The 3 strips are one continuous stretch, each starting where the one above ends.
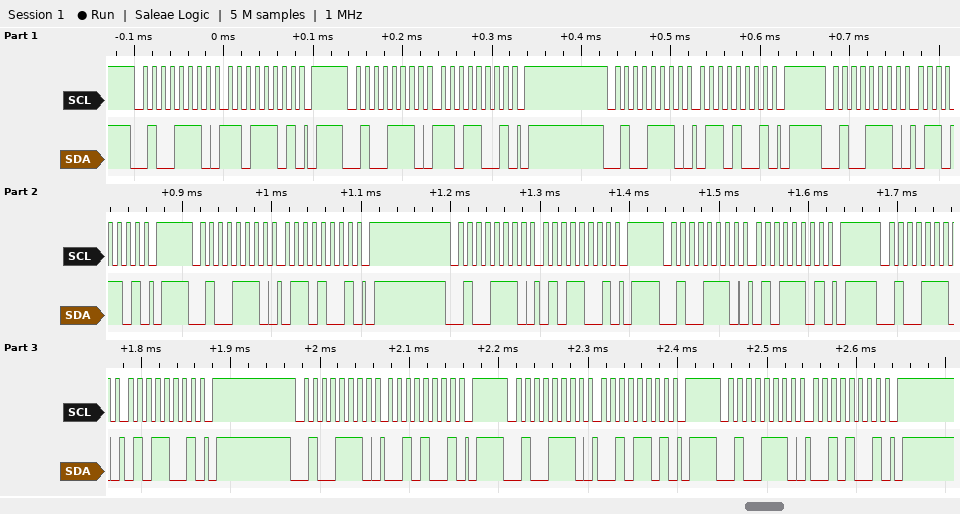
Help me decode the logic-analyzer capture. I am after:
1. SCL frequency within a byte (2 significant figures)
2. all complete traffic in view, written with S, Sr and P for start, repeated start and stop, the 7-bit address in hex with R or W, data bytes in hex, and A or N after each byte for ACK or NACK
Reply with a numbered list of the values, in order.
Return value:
1. 100 kHz
2. S 27W A DD A P S 27W A D9 A P S 27W A 69 A P S 27W A 6D A P S 27W A 69 A P S 27W A 59 A P S 27W A 5D A P S 27W A 59 A P S 27W A 29 A P S 27W A 2D A P S 27W A 29 A P
